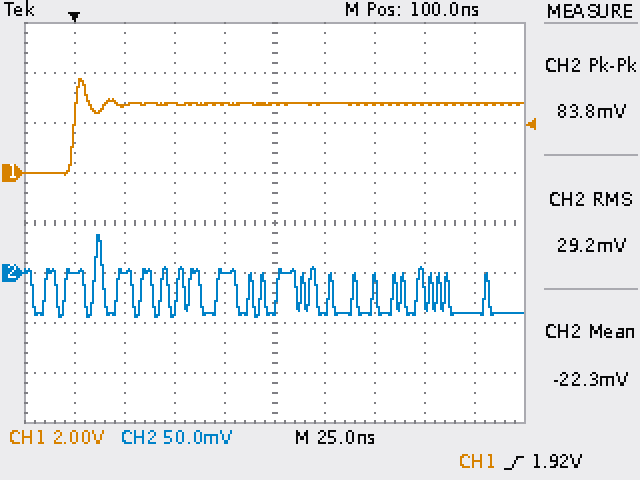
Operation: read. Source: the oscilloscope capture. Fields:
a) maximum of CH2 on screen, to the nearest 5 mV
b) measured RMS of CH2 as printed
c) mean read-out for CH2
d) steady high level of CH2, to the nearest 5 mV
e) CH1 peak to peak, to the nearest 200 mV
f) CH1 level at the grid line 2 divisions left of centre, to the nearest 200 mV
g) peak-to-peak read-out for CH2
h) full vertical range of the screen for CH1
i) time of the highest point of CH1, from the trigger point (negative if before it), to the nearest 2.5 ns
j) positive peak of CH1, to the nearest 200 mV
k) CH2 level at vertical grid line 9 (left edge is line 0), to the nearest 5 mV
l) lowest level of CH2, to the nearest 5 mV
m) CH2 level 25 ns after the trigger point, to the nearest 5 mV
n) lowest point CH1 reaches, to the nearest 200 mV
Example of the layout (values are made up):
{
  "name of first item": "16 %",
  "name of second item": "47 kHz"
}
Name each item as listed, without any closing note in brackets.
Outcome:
{
  "maximum of CH2 on screen, to the nearest 5 mV": "40 mV",
  "measured RMS of CH2 as printed": "29.2 mV",
  "mean read-out for CH2": "-22.3 mV",
  "steady high level of CH2, to the nearest 5 mV": "0 mV",
  "CH1 peak to peak, to the nearest 200 mV": "3.8 V",
  "CH1 level at the grid line 2 divisions left of centre, to the nearest 200 mV": "2.8 V",
  "peak-to-peak read-out for CH2": "83.8 mV",
  "full vertical range of the screen for CH1": "16 V",
  "time of the highest point of CH1, from the trigger point (negative if before it), to the nearest 2.5 ns": "+2.5 ns",
  "positive peak of CH1, to the nearest 200 mV": "3.8 V",
  "CH2 level at vertical grid line 9 (left edge is line 0), to the nearest 5 mV": "-40 mV",
  "lowest level of CH2, to the nearest 5 mV": "-45 mV",
  "CH2 level 25 ns after the trigger point, to the nearest 5 mV": "0 mV",
  "lowest point CH1 reaches, to the nearest 200 mV": "0.0 V"
}
